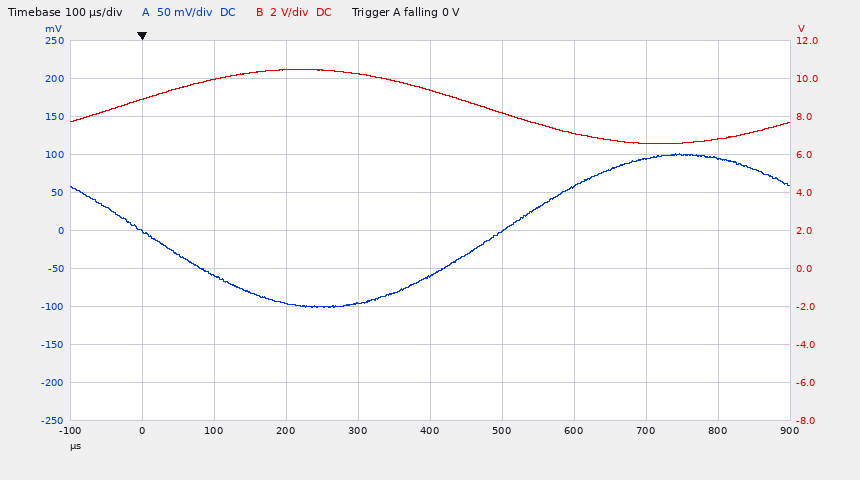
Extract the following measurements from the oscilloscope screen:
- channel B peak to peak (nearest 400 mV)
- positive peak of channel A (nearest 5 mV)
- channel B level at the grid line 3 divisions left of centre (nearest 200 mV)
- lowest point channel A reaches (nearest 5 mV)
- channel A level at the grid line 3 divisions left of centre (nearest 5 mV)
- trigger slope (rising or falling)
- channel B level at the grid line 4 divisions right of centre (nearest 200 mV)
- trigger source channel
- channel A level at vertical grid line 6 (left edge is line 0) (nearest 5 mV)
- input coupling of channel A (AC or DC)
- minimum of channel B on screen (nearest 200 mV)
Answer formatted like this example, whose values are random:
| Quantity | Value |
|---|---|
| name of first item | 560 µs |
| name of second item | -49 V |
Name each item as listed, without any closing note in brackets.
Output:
| Quantity | Value |
|---|---|
| channel B peak to peak | 4.0 V |
| positive peak of channel A | 100 mV |
| channel B level at the grid line 3 divisions left of centre | 10.0 V |
| lowest point channel A reaches | -100 mV |
| channel A level at the grid line 3 divisions left of centre | -60 mV |
| trigger slope | falling |
| channel B level at the grid line 4 divisions right of centre | 6.8 V |
| trigger source channel | channel A |
| channel A level at vertical grid line 6 (left edge is line 0) | 0 mV |
| input coupling of channel A | DC |
| minimum of channel B on screen | 6.6 V |
